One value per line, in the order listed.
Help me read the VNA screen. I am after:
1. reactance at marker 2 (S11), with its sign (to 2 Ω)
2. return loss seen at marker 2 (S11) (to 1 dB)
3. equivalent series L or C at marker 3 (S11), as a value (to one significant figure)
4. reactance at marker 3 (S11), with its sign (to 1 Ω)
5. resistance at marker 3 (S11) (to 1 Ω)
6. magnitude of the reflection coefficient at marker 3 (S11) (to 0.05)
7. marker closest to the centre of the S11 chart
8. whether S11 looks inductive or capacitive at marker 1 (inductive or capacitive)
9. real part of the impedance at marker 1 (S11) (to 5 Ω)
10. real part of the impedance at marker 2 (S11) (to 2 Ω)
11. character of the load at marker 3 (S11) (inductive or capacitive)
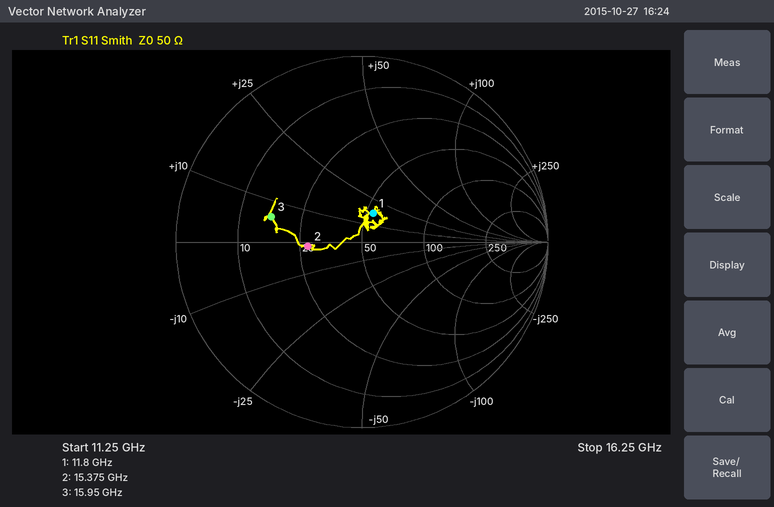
-2 Ω
11 dB
60 pH
+6 Ω
17 Ω
0.50
marker 1
inductive
55 Ω
28 Ω
inductive
